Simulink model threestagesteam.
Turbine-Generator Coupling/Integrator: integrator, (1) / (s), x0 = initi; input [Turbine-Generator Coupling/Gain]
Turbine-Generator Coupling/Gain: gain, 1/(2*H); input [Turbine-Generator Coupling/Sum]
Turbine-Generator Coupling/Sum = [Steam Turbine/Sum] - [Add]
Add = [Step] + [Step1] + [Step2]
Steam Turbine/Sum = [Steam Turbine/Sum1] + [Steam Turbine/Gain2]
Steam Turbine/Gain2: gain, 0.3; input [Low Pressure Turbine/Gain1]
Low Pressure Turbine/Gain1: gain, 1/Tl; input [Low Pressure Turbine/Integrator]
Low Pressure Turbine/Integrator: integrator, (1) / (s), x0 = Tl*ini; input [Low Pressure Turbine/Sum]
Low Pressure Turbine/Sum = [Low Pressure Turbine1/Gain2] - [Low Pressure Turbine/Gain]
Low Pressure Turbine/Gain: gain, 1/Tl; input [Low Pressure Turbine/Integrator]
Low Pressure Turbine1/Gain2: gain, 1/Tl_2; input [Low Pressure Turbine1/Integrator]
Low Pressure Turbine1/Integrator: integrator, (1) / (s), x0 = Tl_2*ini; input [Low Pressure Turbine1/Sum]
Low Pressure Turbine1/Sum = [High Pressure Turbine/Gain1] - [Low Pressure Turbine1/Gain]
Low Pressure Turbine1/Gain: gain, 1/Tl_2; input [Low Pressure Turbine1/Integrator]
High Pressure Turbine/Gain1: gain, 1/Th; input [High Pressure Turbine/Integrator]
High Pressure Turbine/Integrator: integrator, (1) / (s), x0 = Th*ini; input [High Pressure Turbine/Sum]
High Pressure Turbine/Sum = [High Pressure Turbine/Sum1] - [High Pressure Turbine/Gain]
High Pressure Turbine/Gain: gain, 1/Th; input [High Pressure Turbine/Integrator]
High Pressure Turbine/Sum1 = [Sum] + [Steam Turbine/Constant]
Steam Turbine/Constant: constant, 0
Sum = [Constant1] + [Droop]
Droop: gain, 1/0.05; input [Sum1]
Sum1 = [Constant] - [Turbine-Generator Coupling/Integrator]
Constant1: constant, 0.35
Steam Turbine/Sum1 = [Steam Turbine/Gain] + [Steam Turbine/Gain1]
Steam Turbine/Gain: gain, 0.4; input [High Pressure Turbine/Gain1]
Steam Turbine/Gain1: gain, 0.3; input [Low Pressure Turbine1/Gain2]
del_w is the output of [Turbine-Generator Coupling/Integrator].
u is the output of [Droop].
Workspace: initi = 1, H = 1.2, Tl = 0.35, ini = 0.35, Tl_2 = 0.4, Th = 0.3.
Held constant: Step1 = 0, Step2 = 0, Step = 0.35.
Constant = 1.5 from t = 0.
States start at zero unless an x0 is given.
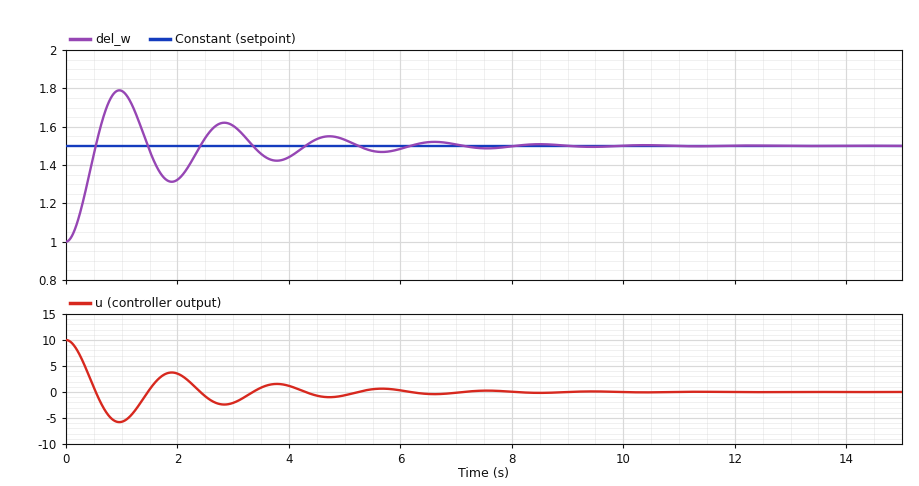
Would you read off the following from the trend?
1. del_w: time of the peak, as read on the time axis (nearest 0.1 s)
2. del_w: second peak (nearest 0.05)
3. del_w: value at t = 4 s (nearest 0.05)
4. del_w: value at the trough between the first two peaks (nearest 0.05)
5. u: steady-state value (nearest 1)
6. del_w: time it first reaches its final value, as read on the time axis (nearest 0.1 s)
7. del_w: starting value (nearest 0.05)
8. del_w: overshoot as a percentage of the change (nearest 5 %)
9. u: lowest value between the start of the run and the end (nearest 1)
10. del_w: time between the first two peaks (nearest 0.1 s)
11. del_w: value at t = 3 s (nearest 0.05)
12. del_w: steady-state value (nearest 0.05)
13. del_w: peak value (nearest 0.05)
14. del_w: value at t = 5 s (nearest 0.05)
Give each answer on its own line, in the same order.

1.0 s
1.60
1.45
1.30
0
0.5 s
1.00
60 %
-6
1.9 s
1.60
1.50
1.80
1.55
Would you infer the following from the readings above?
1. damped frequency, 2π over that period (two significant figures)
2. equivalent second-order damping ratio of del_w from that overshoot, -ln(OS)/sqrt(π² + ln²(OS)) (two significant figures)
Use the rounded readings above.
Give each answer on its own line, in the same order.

3.3 rad/s
0.16
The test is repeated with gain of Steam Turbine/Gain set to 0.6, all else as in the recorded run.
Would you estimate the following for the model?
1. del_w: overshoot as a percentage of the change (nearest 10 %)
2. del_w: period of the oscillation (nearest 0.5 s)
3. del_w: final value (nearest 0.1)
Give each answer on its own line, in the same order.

50 %
1.5 s
1.5
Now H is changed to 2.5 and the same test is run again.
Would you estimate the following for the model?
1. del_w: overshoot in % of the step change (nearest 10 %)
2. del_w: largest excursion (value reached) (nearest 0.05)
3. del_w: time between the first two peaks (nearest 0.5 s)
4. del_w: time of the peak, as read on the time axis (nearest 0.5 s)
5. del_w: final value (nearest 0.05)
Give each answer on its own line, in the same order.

40 %
1.70
2.5 s
1.5 s
1.50
